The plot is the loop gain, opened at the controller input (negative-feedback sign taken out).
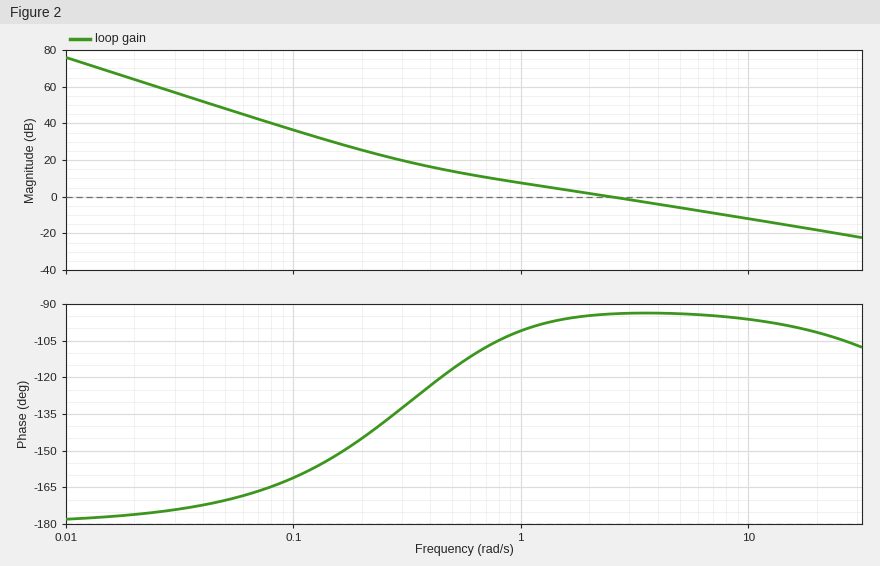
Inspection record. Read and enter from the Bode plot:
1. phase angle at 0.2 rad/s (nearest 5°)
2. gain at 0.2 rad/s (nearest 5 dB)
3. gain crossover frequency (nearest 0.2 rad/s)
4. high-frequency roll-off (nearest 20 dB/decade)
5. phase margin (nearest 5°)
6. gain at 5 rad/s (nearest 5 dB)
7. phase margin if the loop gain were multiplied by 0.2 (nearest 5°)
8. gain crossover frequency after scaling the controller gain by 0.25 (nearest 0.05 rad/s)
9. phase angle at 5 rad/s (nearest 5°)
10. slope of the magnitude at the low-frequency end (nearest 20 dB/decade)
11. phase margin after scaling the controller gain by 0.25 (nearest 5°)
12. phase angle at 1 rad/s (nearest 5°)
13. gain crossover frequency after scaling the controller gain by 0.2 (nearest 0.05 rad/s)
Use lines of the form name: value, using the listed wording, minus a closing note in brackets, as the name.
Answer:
phase angle at 0.2 rad/s: -145°
gain at 0.2 rad/s: 25 dB
gain crossover frequency: 2.4 rad/s
high-frequency roll-off: -20 dB/decade
phase margin: 85°
gain at 5 rad/s: -5 dB
phase margin if the loop gain were multiplied by 0.2: 65°
gain crossover frequency after scaling the controller gain by 0.25: 0.60 rad/s
phase angle at 5 rad/s: -95°
slope of the magnitude at the low-frequency end: -40 dB/decade
phase margin after scaling the controller gain by 0.25: 70°
phase angle at 1 rad/s: -100°
gain crossover frequency after scaling the controller gain by 0.2: 0.50 rad/s
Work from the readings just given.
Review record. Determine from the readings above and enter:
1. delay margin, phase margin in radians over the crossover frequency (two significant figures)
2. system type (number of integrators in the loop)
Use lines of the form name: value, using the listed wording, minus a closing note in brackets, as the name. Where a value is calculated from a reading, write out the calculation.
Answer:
delay margin, phase margin in radians over the crossover frequency: 85 × π / 180 / 2.4 = 0.62 s
system type: 2
